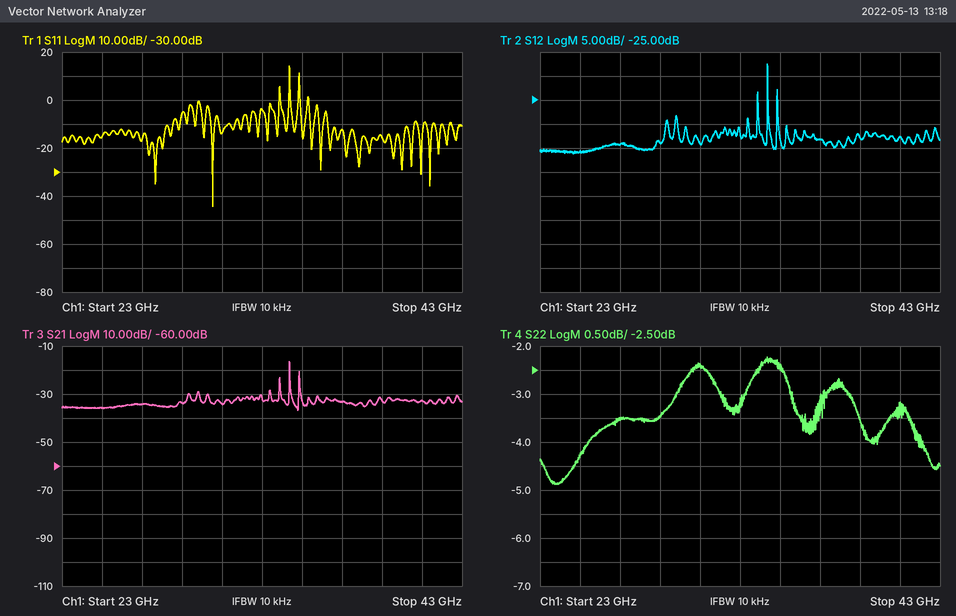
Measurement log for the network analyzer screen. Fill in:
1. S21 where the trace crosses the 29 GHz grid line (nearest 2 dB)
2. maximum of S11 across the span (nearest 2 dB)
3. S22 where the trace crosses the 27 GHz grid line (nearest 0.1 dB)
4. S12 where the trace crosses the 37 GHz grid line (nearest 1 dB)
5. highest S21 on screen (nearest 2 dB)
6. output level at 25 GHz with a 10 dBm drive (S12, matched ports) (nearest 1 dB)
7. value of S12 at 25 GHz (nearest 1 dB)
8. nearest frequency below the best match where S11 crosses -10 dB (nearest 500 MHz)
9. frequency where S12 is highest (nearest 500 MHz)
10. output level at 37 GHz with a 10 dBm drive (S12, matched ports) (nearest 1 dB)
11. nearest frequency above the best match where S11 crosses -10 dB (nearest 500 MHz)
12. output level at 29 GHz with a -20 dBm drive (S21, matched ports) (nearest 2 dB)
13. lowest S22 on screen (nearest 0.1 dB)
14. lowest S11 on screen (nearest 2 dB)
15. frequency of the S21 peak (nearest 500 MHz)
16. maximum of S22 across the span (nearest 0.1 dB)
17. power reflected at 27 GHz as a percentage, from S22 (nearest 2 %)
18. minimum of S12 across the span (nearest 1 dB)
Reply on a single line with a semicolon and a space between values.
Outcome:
-34 dB; 14 dB; -3.5 dB; -33 dB; -16 dB; -26 dBm; -36 dB; 30.5 GHz; 34.5 GHz; -23 dBm; 30.5 GHz; -54 dBm; -4.9 dB; -44 dB; 34.5 GHz; -2.2 dB; 44 %; -36 dB
